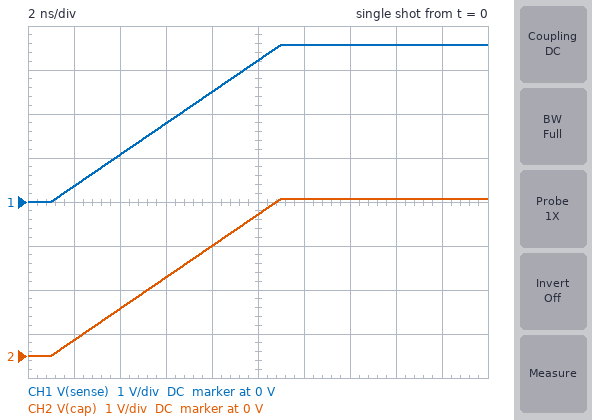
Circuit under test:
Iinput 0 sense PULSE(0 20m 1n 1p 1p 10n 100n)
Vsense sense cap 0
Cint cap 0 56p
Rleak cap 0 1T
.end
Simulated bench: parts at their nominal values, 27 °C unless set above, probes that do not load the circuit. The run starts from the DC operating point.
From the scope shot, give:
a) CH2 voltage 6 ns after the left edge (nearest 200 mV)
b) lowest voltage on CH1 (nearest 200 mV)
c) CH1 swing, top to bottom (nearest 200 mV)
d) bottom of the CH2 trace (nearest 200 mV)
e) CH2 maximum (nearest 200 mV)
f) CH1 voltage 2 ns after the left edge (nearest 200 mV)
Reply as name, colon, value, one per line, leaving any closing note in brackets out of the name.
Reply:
CH2 voltage 6 ns after the left edge: 1.8 V
lowest voltage on CH1: 0 V
CH1 swing, top to bottom: 3.6 V
bottom of the CH2 trace: 0 V
CH2 maximum: 3.6 V
CH1 voltage 2 ns after the left edge: 400 mV
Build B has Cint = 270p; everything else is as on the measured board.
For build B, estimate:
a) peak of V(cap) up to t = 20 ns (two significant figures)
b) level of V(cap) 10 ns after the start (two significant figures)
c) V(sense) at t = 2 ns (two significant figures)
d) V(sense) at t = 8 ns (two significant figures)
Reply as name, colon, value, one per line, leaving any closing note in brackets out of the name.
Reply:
peak of V(cap) up to t = 20 ns: 740 mV
level of V(cap) 10 ns after the start: 670 mV
V(sense) at t = 2 ns: 74 mV
V(sense) at t = 8 ns: 520 mV
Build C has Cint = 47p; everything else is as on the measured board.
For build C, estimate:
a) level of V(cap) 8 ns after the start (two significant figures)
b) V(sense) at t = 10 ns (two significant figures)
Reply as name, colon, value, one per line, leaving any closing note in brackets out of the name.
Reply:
level of V(cap) 8 ns after the start: 3.0 V
V(sense) at t = 10 ns: 3.8 V
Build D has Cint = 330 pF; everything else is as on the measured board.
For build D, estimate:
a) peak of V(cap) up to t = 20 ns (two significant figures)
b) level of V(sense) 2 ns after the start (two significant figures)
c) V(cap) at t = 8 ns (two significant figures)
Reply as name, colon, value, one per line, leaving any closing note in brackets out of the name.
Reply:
peak of V(cap) up to t = 20 ns: 610 mV
level of V(sense) 2 ns after the start: 61 mV
V(cap) at t = 8 ns: 420 mV
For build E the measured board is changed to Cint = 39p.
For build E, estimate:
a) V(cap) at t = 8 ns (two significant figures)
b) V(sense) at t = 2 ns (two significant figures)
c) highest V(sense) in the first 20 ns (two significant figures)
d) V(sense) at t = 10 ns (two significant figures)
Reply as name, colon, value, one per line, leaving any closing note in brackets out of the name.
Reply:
V(cap) at t = 8 ns: 3.6 V
V(sense) at t = 2 ns: 510 mV
highest V(sense) in the first 20 ns: 5.1 V
V(sense) at t = 10 ns: 4.6 V
